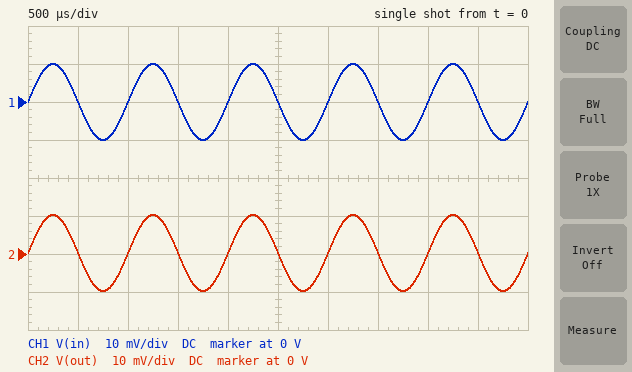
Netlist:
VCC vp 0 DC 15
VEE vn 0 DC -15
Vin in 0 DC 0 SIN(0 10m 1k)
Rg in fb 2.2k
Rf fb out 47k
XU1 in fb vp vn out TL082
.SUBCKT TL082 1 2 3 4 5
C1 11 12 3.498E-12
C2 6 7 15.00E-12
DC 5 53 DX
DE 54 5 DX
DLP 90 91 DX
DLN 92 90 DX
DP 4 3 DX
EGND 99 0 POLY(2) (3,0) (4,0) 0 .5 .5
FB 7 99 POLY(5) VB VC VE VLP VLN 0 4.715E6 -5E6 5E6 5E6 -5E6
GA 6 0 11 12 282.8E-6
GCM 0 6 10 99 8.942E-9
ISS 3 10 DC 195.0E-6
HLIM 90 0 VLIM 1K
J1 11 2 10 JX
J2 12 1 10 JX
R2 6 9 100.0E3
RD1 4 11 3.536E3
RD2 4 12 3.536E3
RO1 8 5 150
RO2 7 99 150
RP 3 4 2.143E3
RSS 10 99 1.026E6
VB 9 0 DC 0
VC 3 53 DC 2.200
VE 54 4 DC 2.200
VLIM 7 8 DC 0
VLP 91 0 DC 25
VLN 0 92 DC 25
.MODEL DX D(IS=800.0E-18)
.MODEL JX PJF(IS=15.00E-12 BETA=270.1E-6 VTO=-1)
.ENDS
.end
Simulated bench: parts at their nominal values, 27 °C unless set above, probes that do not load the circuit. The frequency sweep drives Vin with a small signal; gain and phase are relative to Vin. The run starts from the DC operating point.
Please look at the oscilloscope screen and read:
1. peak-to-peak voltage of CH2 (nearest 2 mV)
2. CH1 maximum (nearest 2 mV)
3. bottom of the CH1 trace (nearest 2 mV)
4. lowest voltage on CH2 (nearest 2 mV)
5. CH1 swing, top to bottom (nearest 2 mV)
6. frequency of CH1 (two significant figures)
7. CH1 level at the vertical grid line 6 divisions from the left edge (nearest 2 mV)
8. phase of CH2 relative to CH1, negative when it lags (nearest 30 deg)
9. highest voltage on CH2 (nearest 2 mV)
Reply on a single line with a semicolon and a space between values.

20 mV; 10 mV; -10 mV; -10 mV; 20 mV; 1.0 kHz; 0 V; 0 deg; 10 mV
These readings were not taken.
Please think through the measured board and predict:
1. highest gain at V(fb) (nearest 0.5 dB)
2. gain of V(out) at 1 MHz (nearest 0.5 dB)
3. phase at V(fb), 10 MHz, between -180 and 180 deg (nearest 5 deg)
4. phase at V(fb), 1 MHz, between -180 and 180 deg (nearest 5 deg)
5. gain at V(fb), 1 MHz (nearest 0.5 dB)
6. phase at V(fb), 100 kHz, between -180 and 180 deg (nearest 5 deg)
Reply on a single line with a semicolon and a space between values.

0 dB; -16.5 dB; 0 deg; 0 deg; -0.5 dB; 0 deg
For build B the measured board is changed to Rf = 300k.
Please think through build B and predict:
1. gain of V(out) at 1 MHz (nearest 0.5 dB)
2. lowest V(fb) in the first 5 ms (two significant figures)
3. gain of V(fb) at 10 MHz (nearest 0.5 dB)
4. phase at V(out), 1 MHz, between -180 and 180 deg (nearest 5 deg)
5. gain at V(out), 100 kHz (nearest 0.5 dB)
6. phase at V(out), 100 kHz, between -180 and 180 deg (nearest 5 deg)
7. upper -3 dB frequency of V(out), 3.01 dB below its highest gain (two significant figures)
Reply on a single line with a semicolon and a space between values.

-32.0 dB; -10 mV; 0 dB; -95 deg; -12.5 dB; -75 deg; 25 kHz
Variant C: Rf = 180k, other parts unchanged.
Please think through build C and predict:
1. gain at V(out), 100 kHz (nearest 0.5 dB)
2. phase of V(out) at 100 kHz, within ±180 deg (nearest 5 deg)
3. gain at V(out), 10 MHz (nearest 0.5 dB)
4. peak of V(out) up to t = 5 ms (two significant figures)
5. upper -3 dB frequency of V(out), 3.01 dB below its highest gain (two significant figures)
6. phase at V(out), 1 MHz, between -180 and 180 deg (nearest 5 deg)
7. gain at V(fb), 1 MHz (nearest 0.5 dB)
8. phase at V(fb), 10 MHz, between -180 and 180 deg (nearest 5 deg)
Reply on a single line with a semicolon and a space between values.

-8.5 dB; -70 deg; -56.0 dB; 11 mV; 42 kHz; -95 deg; 0 dB; 0 deg
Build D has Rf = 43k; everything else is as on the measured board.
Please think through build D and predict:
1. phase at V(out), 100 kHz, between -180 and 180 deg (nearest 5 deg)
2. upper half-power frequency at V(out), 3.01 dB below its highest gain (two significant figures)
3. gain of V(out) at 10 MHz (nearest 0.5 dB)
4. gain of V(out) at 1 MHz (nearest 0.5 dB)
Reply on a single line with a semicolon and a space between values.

-30 deg; 170 kHz; -43.5 dB; -15.5 dB
